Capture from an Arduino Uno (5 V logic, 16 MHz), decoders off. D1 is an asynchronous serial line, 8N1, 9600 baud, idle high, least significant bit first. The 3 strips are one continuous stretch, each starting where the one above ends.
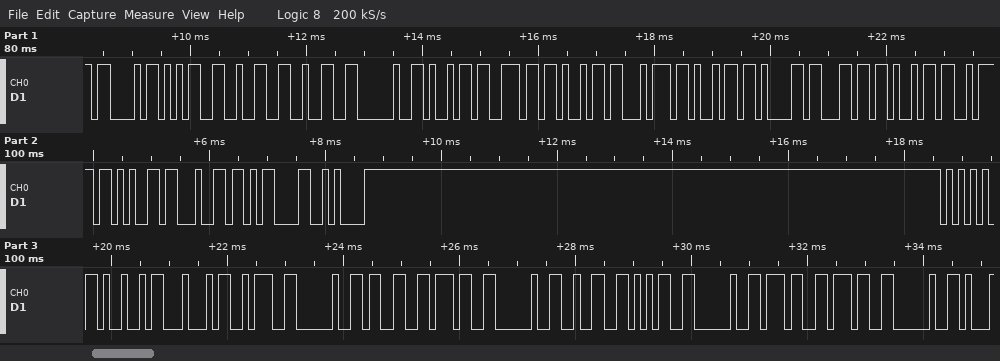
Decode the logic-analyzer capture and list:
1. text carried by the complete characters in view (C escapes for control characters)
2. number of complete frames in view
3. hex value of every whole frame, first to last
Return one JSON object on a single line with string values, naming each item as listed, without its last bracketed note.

{"text carried by the complete characters in view": "\"C522 initialized\\r\\nUID: 37 25 77 \"", "number of complete frames in view": "32", "hex value of every whole frame, first to last": "0x43 0x35 0x32 0x32 0x20 0x69 0x6E 0x69 0x74 0x69 0x61 0x6C 0x69 0x7A 0x65 0x64 0x0D 0x0A 0x55 0x49 0x44 0x3A 0x20 0x33 0x37 0x20 0x32 0x35 0x20 0x37 0x37 0x20"}
